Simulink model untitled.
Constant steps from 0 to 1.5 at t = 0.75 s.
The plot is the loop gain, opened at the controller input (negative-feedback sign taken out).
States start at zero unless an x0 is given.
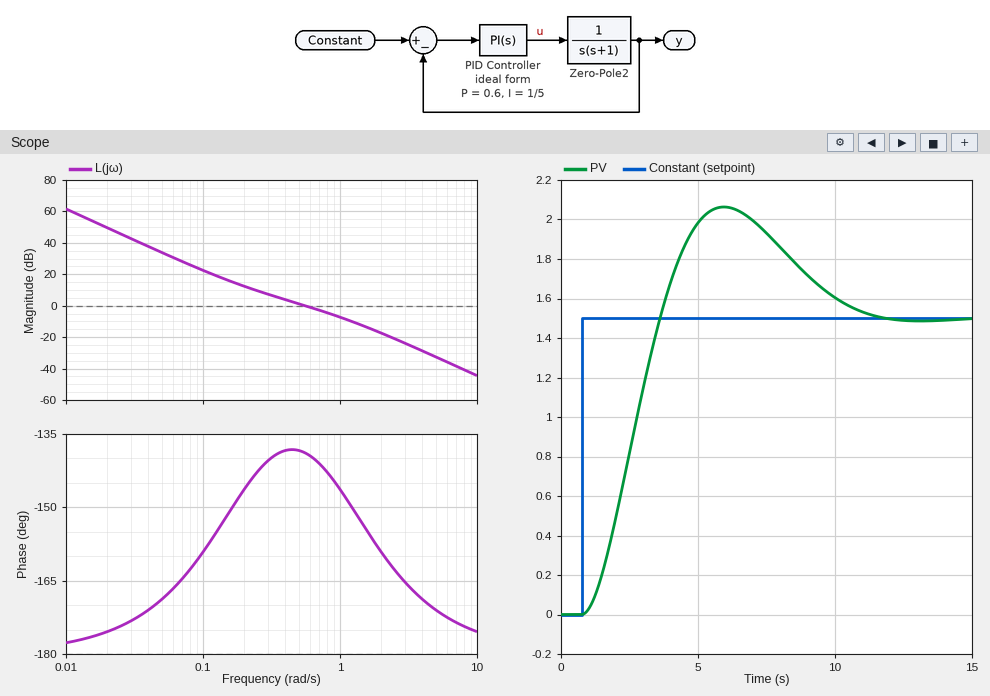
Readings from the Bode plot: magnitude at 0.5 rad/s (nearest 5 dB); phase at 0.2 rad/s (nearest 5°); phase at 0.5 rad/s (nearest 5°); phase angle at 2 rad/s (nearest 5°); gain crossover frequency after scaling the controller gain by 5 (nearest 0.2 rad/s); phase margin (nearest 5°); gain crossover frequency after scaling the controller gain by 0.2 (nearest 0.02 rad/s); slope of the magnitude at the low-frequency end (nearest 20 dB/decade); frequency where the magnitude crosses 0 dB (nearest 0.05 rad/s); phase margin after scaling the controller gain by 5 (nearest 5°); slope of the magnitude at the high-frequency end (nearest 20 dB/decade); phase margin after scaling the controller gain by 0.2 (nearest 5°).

0 dB
-145°
-140°
-160°
1.6 rad/s
40°
0.18 rad/s
-40 dB/decade
0.55 rad/s
25°
-40 dB/decade
30°
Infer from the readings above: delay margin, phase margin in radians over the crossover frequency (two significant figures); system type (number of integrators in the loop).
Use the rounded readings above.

1.3 s
2
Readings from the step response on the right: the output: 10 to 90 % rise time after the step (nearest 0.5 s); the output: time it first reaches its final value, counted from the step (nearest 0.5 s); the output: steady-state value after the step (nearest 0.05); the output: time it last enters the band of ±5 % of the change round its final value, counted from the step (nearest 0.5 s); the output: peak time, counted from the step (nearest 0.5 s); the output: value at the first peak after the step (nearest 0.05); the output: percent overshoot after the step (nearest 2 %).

2.0 s
3.0 s
1.50
9.5 s
5.0 s
2.05
38 %
